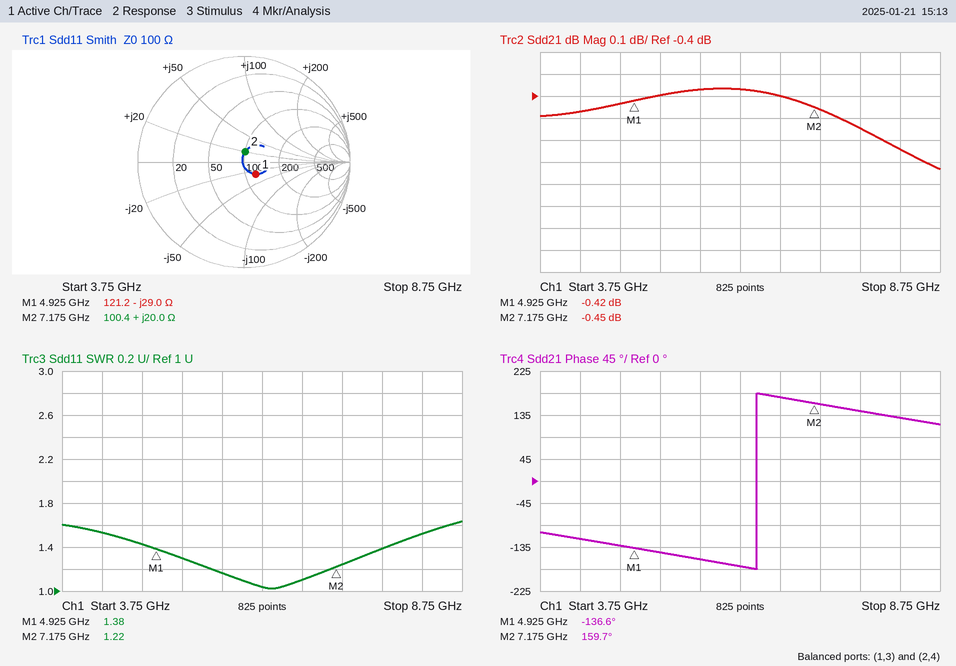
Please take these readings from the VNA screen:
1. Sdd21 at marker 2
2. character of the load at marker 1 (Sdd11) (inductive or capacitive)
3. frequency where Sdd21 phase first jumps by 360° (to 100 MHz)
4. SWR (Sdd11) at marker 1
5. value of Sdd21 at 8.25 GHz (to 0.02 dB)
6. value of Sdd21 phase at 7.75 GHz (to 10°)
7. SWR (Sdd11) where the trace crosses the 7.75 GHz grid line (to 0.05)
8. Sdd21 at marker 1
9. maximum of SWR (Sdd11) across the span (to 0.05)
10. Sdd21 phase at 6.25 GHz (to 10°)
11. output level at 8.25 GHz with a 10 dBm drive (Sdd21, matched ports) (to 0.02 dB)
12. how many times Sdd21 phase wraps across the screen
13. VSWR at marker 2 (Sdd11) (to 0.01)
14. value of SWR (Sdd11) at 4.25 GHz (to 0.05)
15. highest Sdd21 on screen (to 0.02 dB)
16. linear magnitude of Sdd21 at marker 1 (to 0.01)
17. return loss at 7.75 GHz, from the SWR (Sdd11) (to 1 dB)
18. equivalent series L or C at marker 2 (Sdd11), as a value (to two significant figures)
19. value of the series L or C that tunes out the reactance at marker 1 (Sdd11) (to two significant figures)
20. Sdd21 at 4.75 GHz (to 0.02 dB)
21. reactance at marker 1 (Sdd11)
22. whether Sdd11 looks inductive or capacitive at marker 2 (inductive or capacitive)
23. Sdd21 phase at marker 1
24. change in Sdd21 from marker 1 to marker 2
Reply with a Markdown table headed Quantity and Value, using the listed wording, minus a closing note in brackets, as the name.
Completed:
| Quantity | Value |
|---|---|
| Sdd21 at marker 2 | -0.45 dB |
| character of the load at marker 1 (Sdd11) | capacitive |
| frequency where Sdd21 phase first jumps by 360° | 6.5 GHz |
| SWR (Sdd11) at marker 1 | 1.38 |
| value of Sdd21 at 8.25 GHz | -0.64 dB |
| value of Sdd21 phase at 7.75 GHz | 140° |
| SWR (Sdd11) where the trace crosses the 7.75 GHz grid line | 1.40 |
| Sdd21 at marker 1 | -0.42 dB |
| maximum of SWR (Sdd11) across the span | 1.65 |
| Sdd21 phase at 6.25 GHz | -170° |
| output level at 8.25 GHz with a 10 dBm drive (Sdd21, matched ports) | 9.36 dBm |
| how many times Sdd21 phase wraps across the screen | 1 |
| VSWR at marker 2 (Sdd11) | 1.22 |
| value of SWR (Sdd11) at 4.25 GHz | 1.55 |
| highest Sdd21 on screen | -0.36 dB |
| linear magnitude of Sdd21 at marker 1 | 0.95 |
| return loss at 7.75 GHz, from the SWR (Sdd11) | 16 dB |
| equivalent series L or C at marker 2 (Sdd11), as a value | 440 pH |
| value of the series L or C that tunes out the reactance at marker 1 (Sdd11) | 940 pH |
| Sdd21 at 4.75 GHz | -0.44 dB |
| reactance at marker 1 | -29.0 Ω |
| whether Sdd11 looks inductive or capacitive at marker 2 | inductive |
| Sdd21 phase at marker 1 | -136.6° |
| change in Sdd21 from marker 1 to marker 2 | -0.03 dB |
